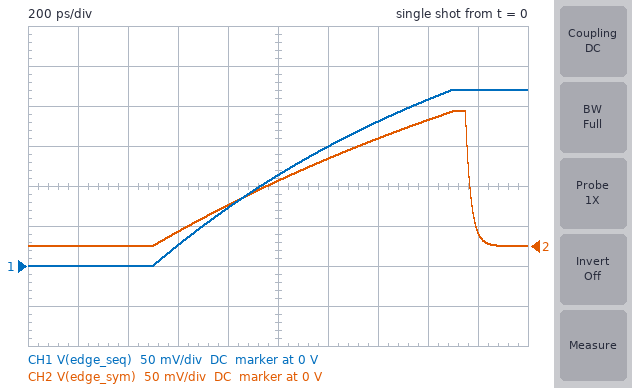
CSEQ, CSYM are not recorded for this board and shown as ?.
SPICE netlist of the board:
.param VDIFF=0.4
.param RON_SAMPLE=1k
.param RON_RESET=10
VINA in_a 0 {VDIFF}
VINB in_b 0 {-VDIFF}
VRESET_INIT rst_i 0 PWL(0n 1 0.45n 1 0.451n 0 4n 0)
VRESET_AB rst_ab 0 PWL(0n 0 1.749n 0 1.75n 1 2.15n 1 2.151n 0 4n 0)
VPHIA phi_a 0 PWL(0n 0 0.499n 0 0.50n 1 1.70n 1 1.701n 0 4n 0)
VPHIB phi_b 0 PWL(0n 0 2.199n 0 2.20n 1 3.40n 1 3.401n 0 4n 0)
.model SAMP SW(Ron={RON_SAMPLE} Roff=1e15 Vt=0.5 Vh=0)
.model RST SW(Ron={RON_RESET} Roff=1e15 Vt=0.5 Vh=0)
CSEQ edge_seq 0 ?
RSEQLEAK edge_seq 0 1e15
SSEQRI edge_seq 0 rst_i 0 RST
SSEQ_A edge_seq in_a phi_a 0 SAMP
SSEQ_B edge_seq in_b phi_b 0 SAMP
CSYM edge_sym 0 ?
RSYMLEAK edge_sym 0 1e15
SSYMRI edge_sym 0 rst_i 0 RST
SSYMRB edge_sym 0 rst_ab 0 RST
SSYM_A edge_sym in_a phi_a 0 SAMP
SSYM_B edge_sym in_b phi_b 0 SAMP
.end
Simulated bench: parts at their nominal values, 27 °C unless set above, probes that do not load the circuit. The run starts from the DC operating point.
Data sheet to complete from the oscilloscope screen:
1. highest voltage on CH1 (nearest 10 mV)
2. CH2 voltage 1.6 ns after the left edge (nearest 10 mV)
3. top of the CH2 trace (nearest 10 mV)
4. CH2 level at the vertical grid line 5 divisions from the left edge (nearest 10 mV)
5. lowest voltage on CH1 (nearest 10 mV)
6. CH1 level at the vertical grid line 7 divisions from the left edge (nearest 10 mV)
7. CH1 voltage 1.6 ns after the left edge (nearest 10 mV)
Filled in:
220 mV
160 mV
170 mV
80 mV
0 V
180 mV
210 mV
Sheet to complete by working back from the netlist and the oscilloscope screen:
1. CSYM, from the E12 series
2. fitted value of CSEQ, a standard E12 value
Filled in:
2.2 pF
1.5 pF
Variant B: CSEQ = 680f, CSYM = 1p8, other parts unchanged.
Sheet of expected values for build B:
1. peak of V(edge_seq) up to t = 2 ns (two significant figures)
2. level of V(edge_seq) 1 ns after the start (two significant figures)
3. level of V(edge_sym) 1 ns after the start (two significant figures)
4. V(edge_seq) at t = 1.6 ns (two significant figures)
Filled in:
330 mV
210 mV
97 mV
320 mV
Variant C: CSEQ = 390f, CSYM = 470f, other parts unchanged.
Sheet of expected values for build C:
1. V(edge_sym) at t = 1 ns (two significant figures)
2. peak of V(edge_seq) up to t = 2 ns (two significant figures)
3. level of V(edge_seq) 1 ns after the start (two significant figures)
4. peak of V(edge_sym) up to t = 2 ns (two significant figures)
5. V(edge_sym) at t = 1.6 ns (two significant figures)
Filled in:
260 mV
380 mV
290 mV
370 mV
360 mV
